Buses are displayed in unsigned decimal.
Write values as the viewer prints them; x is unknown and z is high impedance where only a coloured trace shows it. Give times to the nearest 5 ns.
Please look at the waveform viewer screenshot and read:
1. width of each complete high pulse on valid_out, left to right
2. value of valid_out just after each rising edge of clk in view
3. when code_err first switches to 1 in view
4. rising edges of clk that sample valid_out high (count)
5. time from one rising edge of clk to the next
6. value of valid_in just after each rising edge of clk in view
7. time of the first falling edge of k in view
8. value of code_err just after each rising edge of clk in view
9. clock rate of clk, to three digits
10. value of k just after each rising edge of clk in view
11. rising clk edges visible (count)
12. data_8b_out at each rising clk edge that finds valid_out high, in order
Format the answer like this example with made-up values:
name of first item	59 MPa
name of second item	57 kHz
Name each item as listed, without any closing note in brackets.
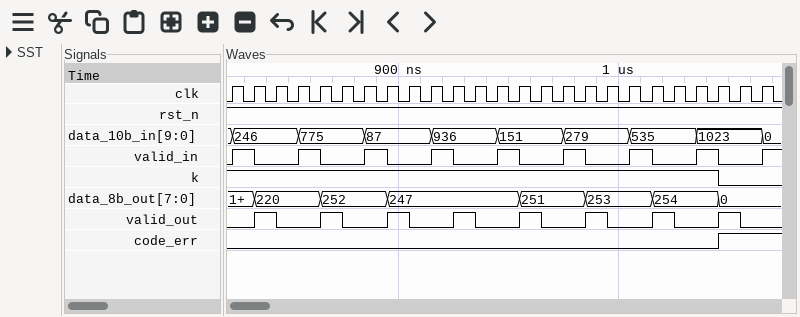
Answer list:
width of each complete high pulse on valid_out, left to right	10 ns, 10 ns, 10 ns, 10 ns, 10 ns, 10 ns, 10 ns, 10 ns
value of valid_out just after each rising edge of clk in view	0 1 0 0 1 0 0 1 0 0 1 0 0 1 0 0 1 0 0 1 0 0 1 0 0
when code_err first switches to 1 in view	1045 ns
rising edges of clk that sample valid_out high	8
time from one rising edge of clk to the next	10 ns
value of valid_in just after each rising edge of clk in view	1 0 0 1 0 0 1 0 0 1 0 0 1 0 0 1 0 0 1 0 0 1 0 0 1
time of the first falling edge of k in view	1045 ns
value of code_err just after each rising edge of clk in view	0 0 0 0 0 0 0 0 0 0 0 0 0 0 0 0 0 0 0 0 0 0 1 1 1
clock rate of clk, to three digits	100 MHz
value of k just after each rising edge of clk in view	1 1 1 1 1 1 1 1 1 1 1 1 1 1 1 1 1 1 1 1 1 1 0 0 0
rising clk edges visible	25
data_8b_out at each rising clk edge that finds valid_out high, in order	220, 252, 247, 247, 251, 253, 254, 0
